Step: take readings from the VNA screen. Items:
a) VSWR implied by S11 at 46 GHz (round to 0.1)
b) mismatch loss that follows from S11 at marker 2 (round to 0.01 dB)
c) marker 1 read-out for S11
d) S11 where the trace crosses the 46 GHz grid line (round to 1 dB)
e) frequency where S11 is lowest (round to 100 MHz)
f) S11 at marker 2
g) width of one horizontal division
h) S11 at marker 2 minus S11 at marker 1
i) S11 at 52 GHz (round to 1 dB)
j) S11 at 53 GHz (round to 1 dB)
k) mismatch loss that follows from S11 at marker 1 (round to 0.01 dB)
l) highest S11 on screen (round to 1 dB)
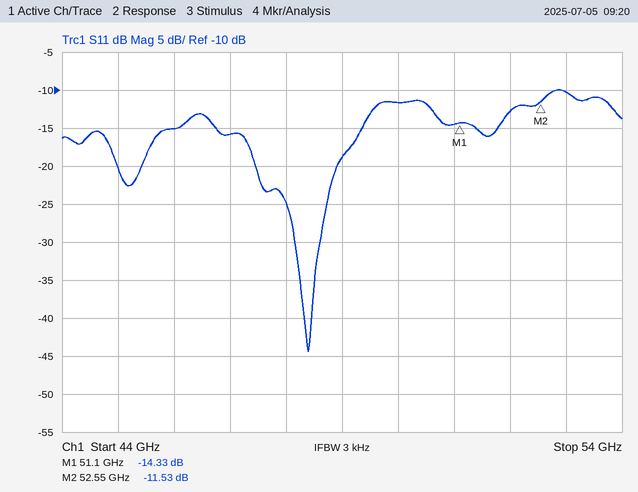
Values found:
1.4
0.32 dB
-14.33 dB
-15 dB
48.4 GHz
-11.53 dB
1 GHz
2.80 dB
-13 dB
-10 dB
0.16 dB
-10 dB
